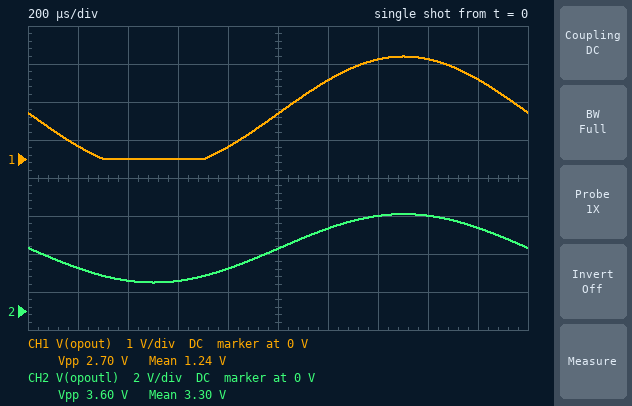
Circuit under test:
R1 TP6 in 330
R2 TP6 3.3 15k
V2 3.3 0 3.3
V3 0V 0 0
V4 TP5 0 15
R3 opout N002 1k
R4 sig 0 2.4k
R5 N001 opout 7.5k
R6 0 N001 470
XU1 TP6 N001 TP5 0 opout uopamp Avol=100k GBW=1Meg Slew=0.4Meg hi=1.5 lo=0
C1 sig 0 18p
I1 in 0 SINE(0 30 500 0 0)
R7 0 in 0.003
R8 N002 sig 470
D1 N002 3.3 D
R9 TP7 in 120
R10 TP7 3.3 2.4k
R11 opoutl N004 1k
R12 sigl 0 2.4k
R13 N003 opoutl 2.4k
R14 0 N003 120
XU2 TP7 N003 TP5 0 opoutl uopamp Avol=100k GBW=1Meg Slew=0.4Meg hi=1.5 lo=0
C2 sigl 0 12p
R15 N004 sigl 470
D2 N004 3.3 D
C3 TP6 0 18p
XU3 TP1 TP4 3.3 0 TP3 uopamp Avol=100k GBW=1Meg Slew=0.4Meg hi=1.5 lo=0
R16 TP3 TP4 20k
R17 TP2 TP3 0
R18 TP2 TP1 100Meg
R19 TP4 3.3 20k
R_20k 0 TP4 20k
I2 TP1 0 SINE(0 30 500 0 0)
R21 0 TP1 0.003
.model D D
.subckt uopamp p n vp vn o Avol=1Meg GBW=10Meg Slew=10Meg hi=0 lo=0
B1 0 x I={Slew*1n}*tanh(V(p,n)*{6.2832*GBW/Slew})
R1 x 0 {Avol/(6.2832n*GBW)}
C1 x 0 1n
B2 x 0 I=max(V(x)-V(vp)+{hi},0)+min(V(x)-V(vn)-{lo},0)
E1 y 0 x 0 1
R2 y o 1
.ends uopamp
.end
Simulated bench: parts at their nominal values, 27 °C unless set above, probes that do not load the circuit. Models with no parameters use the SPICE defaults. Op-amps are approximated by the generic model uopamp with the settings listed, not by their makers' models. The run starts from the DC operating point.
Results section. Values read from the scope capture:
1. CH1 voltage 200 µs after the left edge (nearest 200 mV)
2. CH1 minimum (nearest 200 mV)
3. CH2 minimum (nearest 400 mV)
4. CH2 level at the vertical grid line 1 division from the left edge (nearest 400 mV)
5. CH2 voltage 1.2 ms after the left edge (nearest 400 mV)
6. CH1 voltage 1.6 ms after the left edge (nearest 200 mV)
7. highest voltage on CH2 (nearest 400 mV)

400 mV
0 V
1.6 V
2.4 V
4.4 V
2.6 V
5.2 V
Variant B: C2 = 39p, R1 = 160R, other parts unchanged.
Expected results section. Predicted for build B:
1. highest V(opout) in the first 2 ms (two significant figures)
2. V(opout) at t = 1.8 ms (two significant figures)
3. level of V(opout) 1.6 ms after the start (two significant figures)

2.1 V
1.5 V
2.0 V
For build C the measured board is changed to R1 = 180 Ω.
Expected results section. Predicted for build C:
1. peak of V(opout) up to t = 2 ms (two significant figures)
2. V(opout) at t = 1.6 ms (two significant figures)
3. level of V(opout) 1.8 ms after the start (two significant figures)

2.2 V
2.1 V
1.6 V
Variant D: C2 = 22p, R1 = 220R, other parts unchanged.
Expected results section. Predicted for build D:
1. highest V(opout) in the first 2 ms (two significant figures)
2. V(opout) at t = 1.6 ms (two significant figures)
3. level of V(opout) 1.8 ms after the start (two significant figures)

2.3 V
2.2 V
1.7 V
